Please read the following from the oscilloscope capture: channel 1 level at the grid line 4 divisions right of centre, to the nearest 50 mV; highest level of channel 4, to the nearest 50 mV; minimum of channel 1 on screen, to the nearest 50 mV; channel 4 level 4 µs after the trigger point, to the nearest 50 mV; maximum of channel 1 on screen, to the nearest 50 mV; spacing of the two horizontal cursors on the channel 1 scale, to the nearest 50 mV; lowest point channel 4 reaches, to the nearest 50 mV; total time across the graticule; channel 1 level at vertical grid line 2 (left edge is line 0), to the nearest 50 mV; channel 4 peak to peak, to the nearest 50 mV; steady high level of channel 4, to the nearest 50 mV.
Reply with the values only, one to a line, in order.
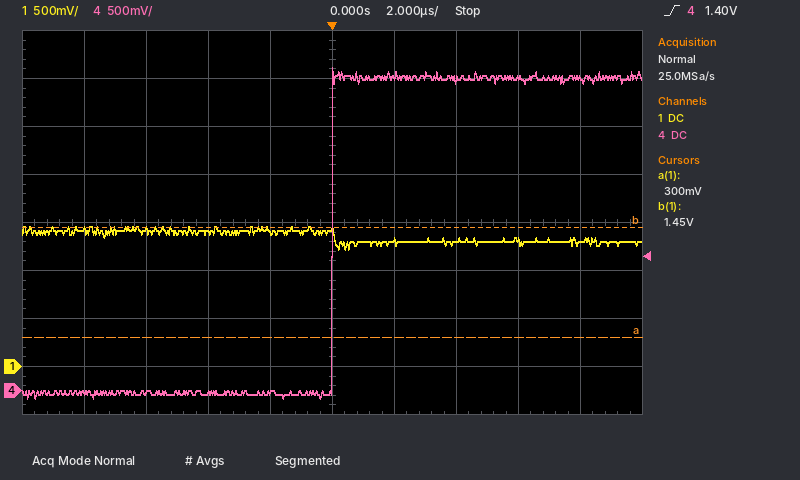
1.30 V
3.35 V
1.20 V
3.25 V
1.45 V
1.15 V
-100 mV
20 µs
1.40 V
3.45 V
3.25 V
